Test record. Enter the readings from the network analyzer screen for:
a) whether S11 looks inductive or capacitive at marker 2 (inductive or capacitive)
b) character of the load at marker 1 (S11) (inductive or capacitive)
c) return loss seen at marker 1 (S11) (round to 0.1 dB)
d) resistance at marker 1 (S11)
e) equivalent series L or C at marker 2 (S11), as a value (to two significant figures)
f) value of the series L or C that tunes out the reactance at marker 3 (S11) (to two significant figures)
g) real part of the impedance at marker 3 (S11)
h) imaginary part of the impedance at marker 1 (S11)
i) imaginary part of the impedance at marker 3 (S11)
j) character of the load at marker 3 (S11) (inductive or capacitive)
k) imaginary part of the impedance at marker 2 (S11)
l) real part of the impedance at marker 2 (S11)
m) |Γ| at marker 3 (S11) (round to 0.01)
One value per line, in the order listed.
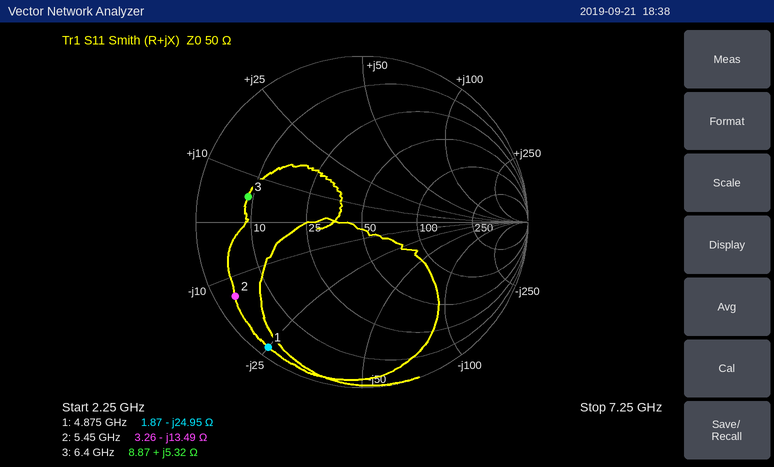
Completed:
capacitive
capacitive
0.5 dB
1.87 Ω
2.2 pF
4.7 pF
8.87 Ω
-24.95 Ω
+5.32 Ω
inductive
-13.49 Ω
3.26 Ω
0.70
